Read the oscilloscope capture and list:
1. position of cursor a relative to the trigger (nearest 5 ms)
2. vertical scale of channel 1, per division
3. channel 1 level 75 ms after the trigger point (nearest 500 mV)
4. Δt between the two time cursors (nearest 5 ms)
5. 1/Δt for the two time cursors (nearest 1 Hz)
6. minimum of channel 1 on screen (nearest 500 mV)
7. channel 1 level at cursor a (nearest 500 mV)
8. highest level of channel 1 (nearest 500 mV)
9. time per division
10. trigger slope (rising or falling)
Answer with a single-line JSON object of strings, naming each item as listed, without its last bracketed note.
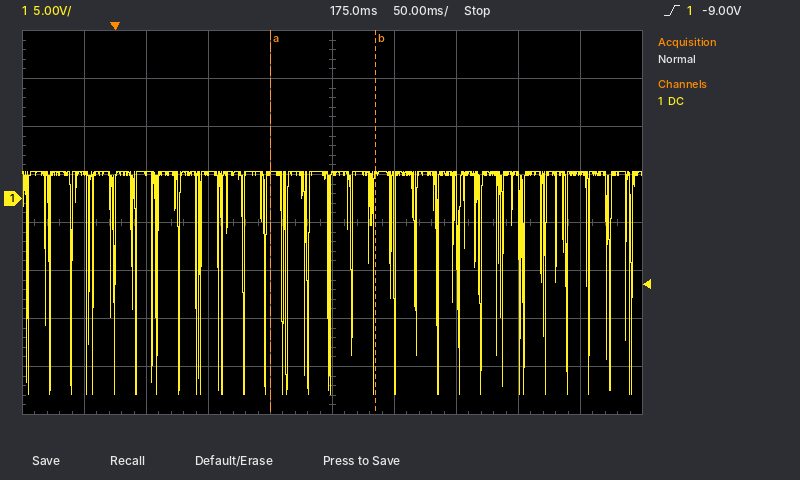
{"position of cursor a relative to the trigger": "+125 ms", "vertical scale of channel 1, per division": "5 V", "channel 1 level 75 ms after the trigger point": "2.5 V", "Δt between the two time cursors": "85 ms", "1/Δt for the two time cursors": "12 Hz", "minimum of channel 1 on screen": "-20.5 V", "channel 1 level at cursor a": "2.5 V", "highest level of channel 1": "3.0 V", "time per division": "50 ms", "trigger slope": "rising"}
